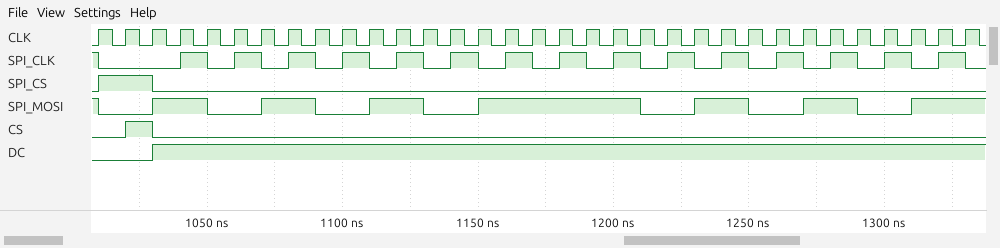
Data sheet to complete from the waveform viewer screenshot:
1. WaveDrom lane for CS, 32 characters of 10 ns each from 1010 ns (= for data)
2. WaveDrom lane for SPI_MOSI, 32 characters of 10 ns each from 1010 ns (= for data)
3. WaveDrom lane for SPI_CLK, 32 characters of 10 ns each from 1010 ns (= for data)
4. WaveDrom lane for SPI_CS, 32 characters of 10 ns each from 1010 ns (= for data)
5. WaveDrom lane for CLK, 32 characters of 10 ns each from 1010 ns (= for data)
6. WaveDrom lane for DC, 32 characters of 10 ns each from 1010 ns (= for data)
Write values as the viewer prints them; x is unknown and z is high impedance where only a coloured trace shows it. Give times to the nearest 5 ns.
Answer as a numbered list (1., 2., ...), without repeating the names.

1. {name: 'CS', wave: '010.............................'}
2. {name: 'SPI_MOSI', wave: '0.1.0.1.0.1.0.1.....0.1.0.1.0.1.'}
3. {name: 'SPI_CLK', wave: '0..10101010101010101010101010101'}
4. {name: 'SPI_CS', wave: '1.0.............................'}
5. {name: 'CLK', wave: 'p...............................'}
6. {name: 'DC', wave: '0.1.............................'}
